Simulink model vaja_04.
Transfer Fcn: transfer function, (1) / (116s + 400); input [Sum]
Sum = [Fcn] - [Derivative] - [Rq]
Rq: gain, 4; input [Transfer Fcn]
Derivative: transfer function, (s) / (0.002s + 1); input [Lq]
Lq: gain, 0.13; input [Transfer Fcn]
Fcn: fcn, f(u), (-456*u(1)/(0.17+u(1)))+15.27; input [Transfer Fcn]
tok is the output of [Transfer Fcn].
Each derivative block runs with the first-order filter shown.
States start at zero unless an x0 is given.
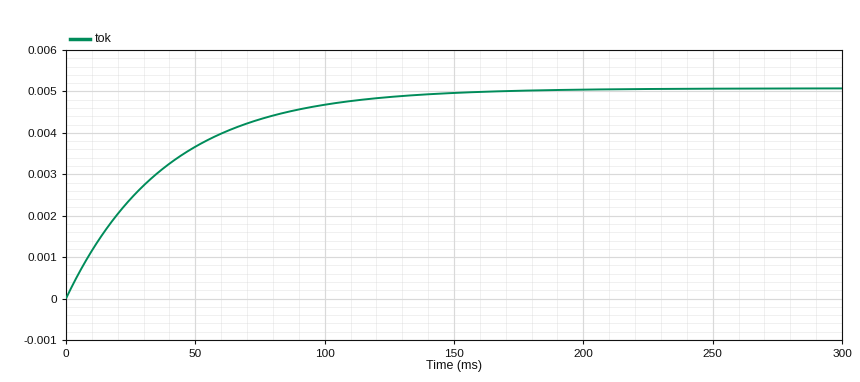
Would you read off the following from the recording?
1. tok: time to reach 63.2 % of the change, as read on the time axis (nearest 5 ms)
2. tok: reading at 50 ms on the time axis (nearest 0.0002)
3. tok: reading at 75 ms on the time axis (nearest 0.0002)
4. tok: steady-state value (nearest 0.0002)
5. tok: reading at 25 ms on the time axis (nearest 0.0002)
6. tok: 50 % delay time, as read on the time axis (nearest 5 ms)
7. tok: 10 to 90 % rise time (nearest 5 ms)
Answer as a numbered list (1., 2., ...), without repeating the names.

1. 40 ms
2. 0.0036
3. 0.0044
4. 0.0050
5. 0.0024
6. 25 ms
7. 85 ms
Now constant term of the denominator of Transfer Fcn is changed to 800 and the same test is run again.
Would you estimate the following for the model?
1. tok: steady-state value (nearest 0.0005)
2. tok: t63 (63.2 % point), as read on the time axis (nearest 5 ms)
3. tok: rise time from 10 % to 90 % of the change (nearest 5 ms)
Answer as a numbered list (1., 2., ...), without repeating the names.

1. 0.0045
2. 35 ms
3. 75 ms
